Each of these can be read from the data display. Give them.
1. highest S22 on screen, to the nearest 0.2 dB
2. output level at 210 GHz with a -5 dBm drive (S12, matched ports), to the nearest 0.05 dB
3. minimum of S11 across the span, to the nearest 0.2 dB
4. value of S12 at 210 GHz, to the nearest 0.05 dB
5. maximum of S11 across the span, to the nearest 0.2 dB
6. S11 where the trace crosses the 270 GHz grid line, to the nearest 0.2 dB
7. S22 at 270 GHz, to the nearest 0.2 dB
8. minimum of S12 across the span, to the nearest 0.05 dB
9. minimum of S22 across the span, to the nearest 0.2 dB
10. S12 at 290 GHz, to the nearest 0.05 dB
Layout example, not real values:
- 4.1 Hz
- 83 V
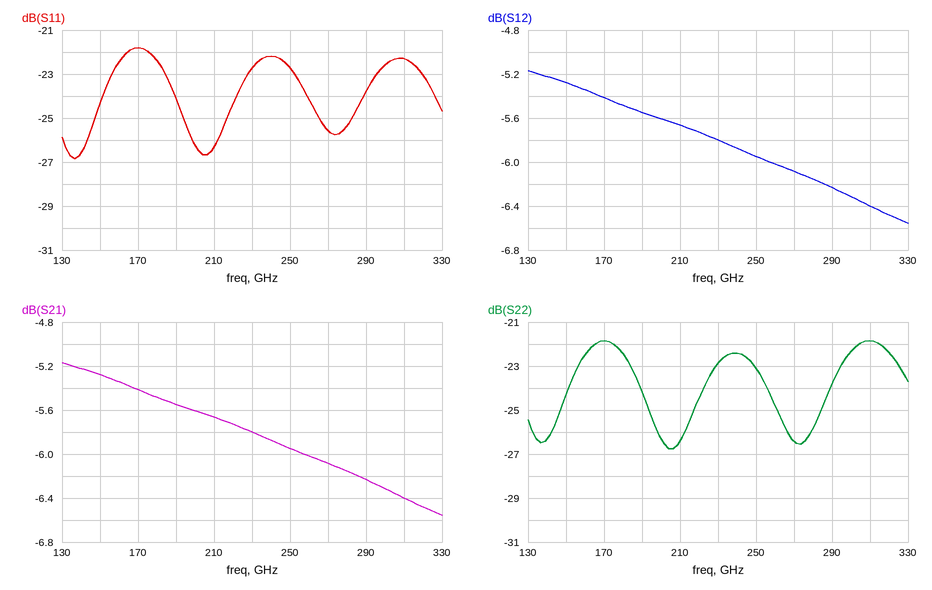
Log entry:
- -21.8 dB
- -10.65 dBm
- -26.8 dB
- -5.65 dB
- -21.8 dB
- -25.6 dB
- -26.4 dB
- -6.55 dB
- -26.8 dB
- -6.25 dB
